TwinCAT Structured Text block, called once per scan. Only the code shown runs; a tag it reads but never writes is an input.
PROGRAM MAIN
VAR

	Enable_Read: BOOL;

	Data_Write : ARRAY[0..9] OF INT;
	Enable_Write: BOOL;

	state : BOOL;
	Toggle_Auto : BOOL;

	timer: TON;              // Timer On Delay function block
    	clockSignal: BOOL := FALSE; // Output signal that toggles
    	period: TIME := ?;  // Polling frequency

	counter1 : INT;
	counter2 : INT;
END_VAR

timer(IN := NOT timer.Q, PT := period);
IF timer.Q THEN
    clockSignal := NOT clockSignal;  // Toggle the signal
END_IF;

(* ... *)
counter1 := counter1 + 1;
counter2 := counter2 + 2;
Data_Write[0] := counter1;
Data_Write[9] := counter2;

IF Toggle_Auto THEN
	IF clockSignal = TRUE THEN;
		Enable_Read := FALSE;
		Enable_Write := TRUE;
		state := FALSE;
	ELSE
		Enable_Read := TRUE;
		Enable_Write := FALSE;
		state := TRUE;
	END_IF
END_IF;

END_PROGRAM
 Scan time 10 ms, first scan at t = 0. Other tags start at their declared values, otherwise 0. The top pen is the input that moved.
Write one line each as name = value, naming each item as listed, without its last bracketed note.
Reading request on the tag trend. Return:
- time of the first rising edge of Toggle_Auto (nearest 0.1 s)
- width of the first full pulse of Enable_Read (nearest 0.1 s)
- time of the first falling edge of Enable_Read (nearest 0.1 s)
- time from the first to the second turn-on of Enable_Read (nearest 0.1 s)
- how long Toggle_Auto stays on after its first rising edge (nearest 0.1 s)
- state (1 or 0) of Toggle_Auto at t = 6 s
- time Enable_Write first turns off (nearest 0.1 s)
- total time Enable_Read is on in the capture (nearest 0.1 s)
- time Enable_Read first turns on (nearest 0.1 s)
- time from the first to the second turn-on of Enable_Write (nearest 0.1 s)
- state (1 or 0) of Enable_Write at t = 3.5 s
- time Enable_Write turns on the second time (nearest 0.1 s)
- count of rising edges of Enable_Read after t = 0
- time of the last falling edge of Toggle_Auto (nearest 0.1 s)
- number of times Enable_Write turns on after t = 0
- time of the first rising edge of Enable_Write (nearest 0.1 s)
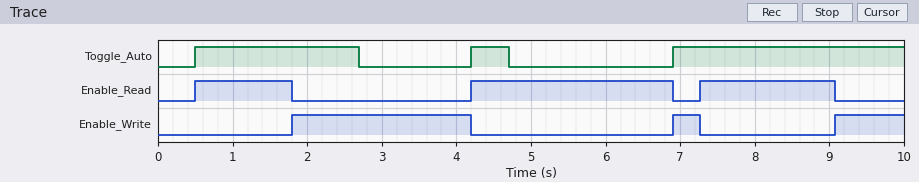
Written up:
time of the first rising edge of Toggle_Auto = 0.5 s
width of the first full pulse of Enable_Read = 1.3 s
time of the first falling edge of Enable_Read = 1.8 s
time from the first to the second turn-on of Enable_Read = 3.7 s
how long Toggle_Auto stays on after its first rising edge = 2.2 s
state (1 or 0) of Toggle_Auto at t = 6 s = 0
time Enable_Write first turns off = 4.2 s
total time Enable_Read is on in the capture = 5.8 s
time Enable_Read first turns on = 0.5 s
time from the first to the second turn-on of Enable_Write = 5.1 s
state (1 or 0) of Enable_Write at t = 3.5 s = 1
time Enable_Write turns on the second time = 6.9 s
count of rising edges of Enable_Read after t = 0 = 3
time of the last falling edge of Toggle_Auto = 4.7 s
number of times Enable_Write turns on after t = 0 = 3
time of the first rising edge of Enable_Write = 1.8 s
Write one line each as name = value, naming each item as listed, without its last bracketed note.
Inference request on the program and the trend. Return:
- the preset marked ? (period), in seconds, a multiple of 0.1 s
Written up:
the preset marked ? (period), in seconds, a multiple of 0.1 s = 1.8 s
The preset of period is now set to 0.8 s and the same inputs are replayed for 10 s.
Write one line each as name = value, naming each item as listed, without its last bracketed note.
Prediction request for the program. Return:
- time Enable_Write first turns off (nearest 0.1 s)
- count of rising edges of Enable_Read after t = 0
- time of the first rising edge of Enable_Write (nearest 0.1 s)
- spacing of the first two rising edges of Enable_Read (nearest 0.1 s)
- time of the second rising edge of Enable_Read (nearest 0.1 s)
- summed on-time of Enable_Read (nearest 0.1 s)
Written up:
time Enable_Write first turns off = 1.6 s
count of rising edges of Enable_Read after t = 0 = 5
time of the first rising edge of Enable_Write = 0.8 s
spacing of the first two rising edges of Enable_Read = 1.1 s
time of the second rising edge of Enable_Read = 1.6 s
summed on-time of Enable_Read = 2.6 s
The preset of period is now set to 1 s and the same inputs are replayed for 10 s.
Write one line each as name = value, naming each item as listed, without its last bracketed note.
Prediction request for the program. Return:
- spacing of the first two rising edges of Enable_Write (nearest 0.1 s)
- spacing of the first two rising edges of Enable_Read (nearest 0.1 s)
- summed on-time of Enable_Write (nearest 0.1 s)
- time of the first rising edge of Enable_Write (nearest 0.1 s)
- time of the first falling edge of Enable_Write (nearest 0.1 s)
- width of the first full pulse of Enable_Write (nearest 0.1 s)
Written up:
spacing of the first two rising edges of Enable_Write = 6.1 s
spacing of the first two rising edges of Enable_Read = 1.5 s
summed on-time of Enable_Write = 2.9 s
time of the first rising edge of Enable_Write = 1.0 s
time of the first falling edge of Enable_Write = 2.0 s
width of the first full pulse of Enable_Write = 1.0 s
